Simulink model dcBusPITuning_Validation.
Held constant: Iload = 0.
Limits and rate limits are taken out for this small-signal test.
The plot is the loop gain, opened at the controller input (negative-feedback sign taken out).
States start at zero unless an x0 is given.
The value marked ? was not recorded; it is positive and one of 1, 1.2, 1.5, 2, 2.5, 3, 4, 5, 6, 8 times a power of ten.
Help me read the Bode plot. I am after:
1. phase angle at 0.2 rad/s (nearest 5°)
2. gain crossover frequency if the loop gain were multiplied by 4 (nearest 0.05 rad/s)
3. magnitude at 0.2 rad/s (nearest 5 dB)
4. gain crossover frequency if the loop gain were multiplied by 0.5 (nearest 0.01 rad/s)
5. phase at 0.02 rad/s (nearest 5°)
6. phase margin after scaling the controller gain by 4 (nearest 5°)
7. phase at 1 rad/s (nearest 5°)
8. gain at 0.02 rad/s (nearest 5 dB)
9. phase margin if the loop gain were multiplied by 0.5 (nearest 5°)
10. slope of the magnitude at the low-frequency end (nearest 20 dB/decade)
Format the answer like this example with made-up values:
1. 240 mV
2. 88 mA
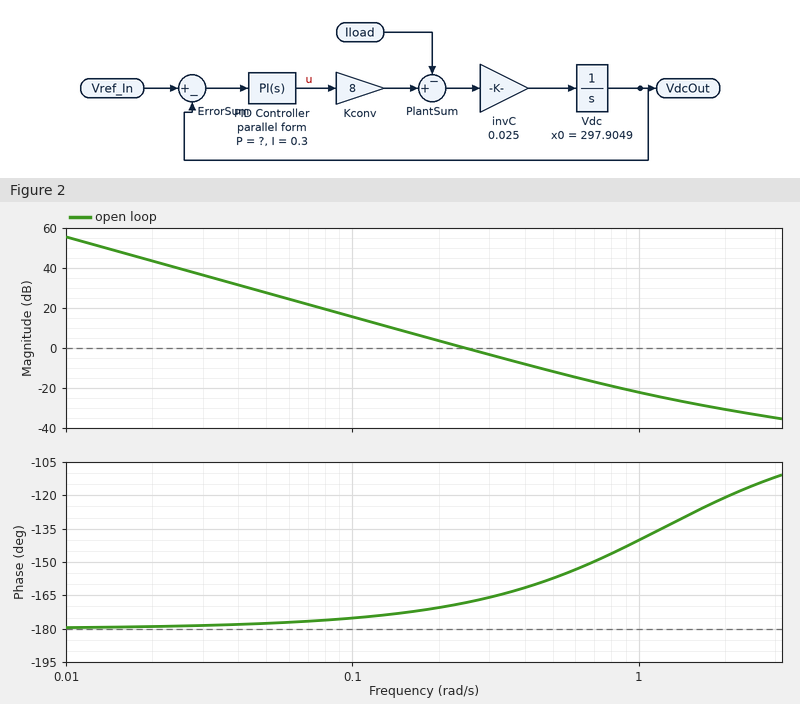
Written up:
1. -170°
2. 0.50 rad/s
3. 5 dB
4. 0.17 rad/s
5. -180°
6. 25°
7. -140°
8. 45 dB
9. 10°
10. -40 dB/decade
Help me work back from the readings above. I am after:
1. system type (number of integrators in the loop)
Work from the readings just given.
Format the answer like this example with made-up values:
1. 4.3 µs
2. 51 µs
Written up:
1. 2
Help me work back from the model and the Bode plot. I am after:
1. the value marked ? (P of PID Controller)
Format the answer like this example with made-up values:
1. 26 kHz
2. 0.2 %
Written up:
1. 0.25
